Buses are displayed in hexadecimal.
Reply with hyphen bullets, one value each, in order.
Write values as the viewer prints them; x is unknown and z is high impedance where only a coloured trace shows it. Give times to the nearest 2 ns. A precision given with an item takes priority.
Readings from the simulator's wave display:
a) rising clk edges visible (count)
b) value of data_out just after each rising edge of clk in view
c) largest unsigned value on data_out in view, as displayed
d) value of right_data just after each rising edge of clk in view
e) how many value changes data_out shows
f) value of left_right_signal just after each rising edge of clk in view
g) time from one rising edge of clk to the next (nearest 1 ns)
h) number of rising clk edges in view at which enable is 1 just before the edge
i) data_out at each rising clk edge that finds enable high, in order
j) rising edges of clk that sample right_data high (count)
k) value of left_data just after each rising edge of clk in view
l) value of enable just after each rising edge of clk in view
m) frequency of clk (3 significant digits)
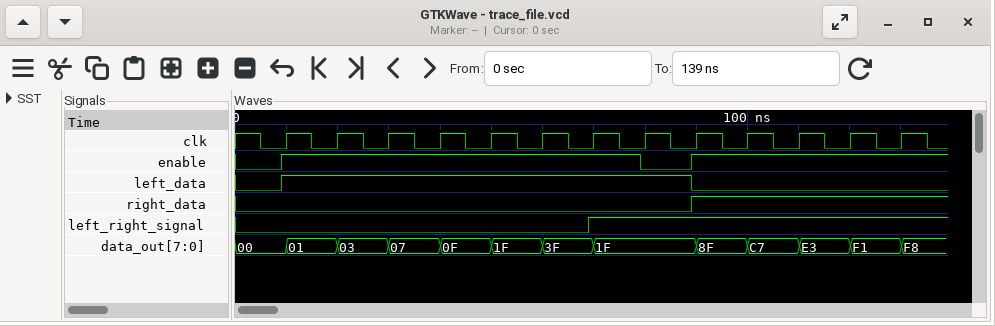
- 13
- 01, 03, 07, 0F, 1F, 3F, 1F, 1F, 8F, C7, E3, F1, F8
- F8
- 0 0 0 0 0 0 0 0 1 1 1 1 1
- 12
- 0 0 0 0 0 0 1 1 1 1 1 1 1
- 10 ns
- 12
- 00, 01, 03, 07, 0F, 1F, 3F, 1F, 8F, C7, E3, F1
- 5
- 1 1 1 1 1 1 1 1 0 0 0 0 0
- 1 1 1 1 1 1 1 0 1 1 1 1 1
- 100 MHz
